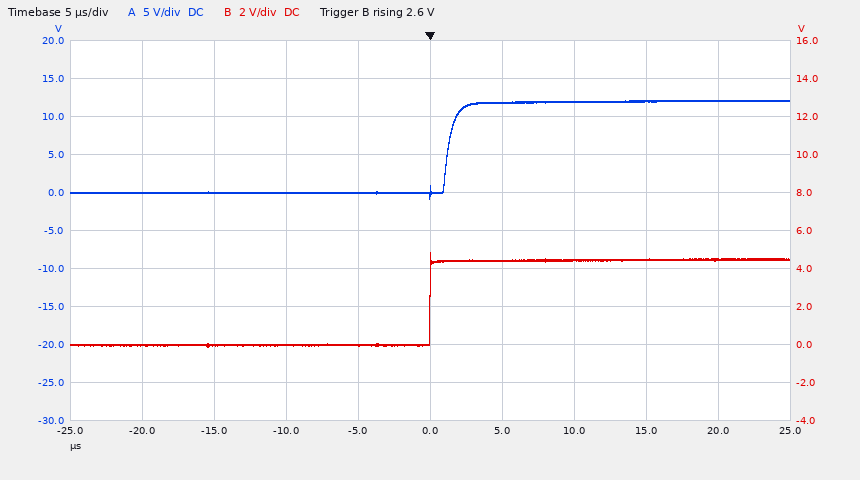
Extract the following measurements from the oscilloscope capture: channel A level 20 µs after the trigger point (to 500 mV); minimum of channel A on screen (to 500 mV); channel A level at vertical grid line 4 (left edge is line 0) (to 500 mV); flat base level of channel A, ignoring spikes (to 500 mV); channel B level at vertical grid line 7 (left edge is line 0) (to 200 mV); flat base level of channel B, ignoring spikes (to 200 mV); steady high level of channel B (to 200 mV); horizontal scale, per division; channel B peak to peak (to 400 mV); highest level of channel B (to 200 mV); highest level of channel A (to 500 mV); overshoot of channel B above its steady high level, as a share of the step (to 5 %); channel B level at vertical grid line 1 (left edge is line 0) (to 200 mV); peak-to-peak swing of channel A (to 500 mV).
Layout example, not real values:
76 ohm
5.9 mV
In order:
12.0 V
-1.0 V
0.0 V
0.0 V
4.4 V
0.0 V
4.4 V
5 µs
4.8 V
4.8 V
12.0 V
10 %
0.0 V
13.0 V
